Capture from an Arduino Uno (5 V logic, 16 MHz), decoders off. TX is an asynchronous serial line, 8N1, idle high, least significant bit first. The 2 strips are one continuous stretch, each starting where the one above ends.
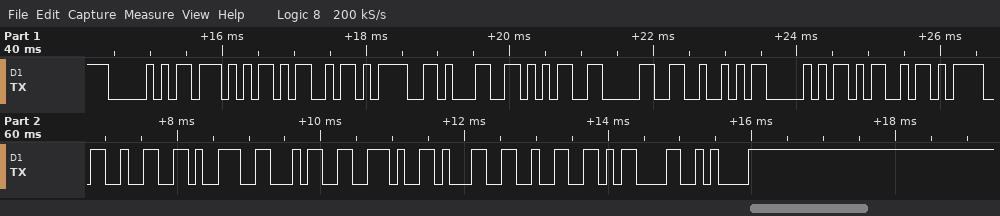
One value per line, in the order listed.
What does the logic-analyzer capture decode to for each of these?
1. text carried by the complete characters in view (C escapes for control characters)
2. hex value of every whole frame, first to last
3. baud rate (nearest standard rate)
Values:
"PWM=150RPM=294.12\r\n"
0x50 0x57 0x4D 0x3D 0x31 0x35 0x30 0x52 0x50 0x4D 0x3D 0x32 0x39 0x34 0x2E 0x31 0x32 0x0D 0x0A
9600 baud
